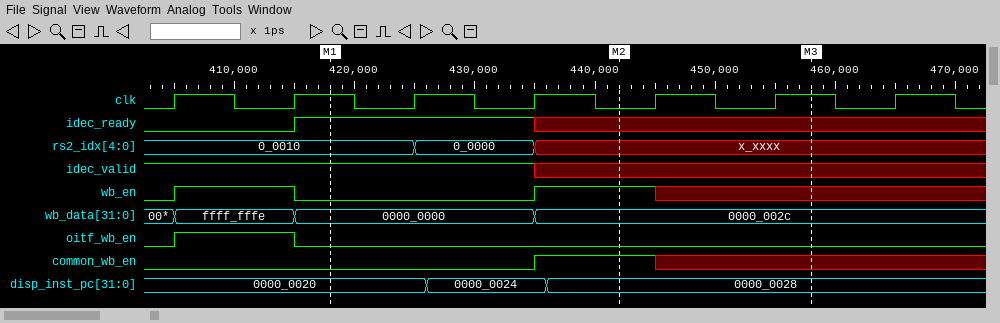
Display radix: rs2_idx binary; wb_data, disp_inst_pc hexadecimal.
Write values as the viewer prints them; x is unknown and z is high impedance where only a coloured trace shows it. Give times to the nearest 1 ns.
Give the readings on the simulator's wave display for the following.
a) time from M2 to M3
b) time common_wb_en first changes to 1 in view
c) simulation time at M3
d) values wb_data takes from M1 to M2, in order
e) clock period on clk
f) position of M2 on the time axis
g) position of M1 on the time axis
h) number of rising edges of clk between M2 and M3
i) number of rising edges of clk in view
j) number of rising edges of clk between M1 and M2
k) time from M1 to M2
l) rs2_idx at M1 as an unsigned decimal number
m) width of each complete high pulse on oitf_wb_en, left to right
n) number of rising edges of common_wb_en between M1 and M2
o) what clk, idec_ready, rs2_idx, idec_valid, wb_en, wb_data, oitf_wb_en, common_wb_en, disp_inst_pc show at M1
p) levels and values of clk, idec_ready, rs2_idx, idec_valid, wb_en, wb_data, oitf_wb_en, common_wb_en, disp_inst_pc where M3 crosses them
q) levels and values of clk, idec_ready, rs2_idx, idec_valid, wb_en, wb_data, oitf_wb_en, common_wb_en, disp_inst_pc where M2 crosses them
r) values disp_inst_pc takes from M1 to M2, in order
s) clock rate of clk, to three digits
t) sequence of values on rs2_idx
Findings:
16 ns
435 ns
458 ns
0000_0000, 0000_002c
10 ns
442 ns
418 ns
2
7
2
24 ns
2
10 ns
1
clk=1, idec_ready=1, rs2_idx=0_0010, idec_valid=1, wb_en=0, wb_data=0000_0000, oitf_wb_en=0, common_wb_en=0, disp_inst_pc=0000_0020
clk=1, idec_ready=x, rs2_idx=x_xxxx, idec_valid=x, wb_en=x, wb_data=0000_002c, oitf_wb_en=0, common_wb_en=x, disp_inst_pc=0000_0028
clk=0, idec_ready=x, rs2_idx=x_xxxx, idec_valid=x, wb_en=1, wb_data=0000_002c, oitf_wb_en=0, common_wb_en=1, disp_inst_pc=0000_0028
0000_0020, 0000_0024, 0000_0028
100 MHz
0_0010, 0_0000, x_xxxx
